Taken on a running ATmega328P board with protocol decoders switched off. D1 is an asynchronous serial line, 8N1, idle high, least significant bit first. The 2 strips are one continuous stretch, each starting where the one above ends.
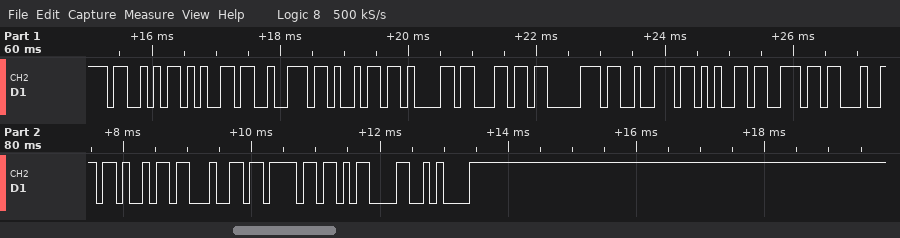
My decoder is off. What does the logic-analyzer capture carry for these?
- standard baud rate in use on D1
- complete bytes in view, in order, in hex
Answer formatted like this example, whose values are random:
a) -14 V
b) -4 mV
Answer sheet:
a) 9600 baud
b) 0x53 0x65 0x72 0x69 0x61 0x6C 0x70 0x72 0x65 0x6E 0x64 0x69 0x64 0x6F 0x0D 0x0A
